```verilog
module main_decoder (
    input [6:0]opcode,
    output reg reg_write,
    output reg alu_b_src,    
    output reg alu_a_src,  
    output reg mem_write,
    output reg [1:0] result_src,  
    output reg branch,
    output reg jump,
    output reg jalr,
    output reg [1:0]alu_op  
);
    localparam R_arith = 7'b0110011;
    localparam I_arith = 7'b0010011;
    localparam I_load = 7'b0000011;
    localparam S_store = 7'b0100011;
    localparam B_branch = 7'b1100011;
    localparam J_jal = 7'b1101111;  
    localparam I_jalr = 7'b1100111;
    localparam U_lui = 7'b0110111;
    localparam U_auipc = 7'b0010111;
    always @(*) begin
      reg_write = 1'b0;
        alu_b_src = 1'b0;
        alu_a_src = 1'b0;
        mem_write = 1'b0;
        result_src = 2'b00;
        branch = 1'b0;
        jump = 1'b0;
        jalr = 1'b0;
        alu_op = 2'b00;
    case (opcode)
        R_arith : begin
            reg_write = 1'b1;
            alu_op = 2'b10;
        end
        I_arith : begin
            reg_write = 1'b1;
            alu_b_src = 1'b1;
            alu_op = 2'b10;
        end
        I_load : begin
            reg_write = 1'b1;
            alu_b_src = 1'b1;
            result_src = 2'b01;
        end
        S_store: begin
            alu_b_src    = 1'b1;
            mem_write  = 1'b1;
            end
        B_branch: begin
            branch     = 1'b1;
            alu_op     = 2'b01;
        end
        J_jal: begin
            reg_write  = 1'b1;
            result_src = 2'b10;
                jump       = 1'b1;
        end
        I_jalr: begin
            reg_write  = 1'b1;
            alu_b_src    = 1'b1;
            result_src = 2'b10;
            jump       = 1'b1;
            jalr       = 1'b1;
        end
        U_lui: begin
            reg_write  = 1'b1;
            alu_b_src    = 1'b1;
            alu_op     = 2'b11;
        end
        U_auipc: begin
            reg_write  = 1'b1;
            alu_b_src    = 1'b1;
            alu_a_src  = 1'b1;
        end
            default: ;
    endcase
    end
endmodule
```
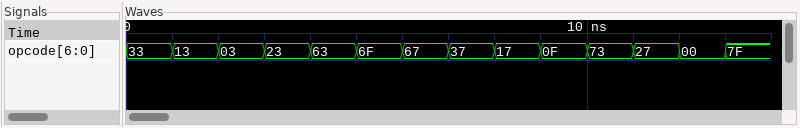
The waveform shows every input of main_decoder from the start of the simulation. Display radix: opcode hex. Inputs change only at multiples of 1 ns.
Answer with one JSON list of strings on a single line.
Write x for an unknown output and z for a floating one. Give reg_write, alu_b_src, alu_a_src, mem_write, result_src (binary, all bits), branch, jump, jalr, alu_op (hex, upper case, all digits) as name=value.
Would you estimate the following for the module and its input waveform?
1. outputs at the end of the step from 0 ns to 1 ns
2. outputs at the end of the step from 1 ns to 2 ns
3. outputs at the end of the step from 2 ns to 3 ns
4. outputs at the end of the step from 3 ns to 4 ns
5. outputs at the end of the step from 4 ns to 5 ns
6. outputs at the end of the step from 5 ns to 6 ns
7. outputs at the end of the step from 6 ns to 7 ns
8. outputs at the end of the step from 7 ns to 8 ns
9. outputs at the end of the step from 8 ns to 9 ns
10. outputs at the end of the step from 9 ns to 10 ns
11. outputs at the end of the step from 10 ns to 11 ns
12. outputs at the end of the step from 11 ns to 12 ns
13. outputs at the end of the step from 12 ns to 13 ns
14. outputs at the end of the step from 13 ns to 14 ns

["reg_write=1, alu_b_src=0, alu_a_src=0, mem_write=0, result_src=00, branch=0, jump=0, jalr=0, alu_op=2", "reg_write=1, alu_b_src=1, alu_a_src=0, mem_write=0, result_src=00, branch=0, jump=0, jalr=0, alu_op=2", "reg_write=1, alu_b_src=1, alu_a_src=0, mem_write=0, result_src=01, branch=0, jump=0, jalr=0, alu_op=0", "reg_write=0, alu_b_src=1, alu_a_src=0, mem_write=1, result_src=00, branch=0, jump=0, jalr=0, alu_op=0", "reg_write=0, alu_b_src=0, alu_a_src=0, mem_write=0, result_src=00, branch=1, jump=0, jalr=0, alu_op=1", "reg_write=1, alu_b_src=0, alu_a_src=0, mem_write=0, result_src=10, branch=0, jump=1, jalr=0, alu_op=0", "reg_write=1, alu_b_src=1, alu_a_src=0, mem_write=0, result_src=10, branch=0, jump=1, jalr=1, alu_op=0", "reg_write=1, alu_b_src=1, alu_a_src=0, mem_write=0, result_src=00, branch=0, jump=0, jalr=0, alu_op=3", "reg_write=1, alu_b_src=1, alu_a_src=1, mem_write=0, result_src=00, branch=0, jump=0, jalr=0, alu_op=0", "reg_write=0, alu_b_src=0, alu_a_src=0, mem_write=0, result_src=00, branch=0, jump=0, jalr=0, alu_op=0", "reg_write=0, alu_b_src=0, alu_a_src=0, mem_write=0, result_src=00, branch=0, jump=0, jalr=0, alu_op=0", "reg_write=0, alu_b_src=0, alu_a_src=0, mem_write=0, result_src=00, branch=0, jump=0, jalr=0, alu_op=0", "reg_write=0, alu_b_src=0, alu_a_src=0, mem_write=0, result_src=00, branch=0, jump=0, jalr=0, alu_op=0", "reg_write=0, alu_b_src=0, alu_a_src=0, mem_write=0, result_src=00, branch=0, jump=0, jalr=0, alu_op=0"]
